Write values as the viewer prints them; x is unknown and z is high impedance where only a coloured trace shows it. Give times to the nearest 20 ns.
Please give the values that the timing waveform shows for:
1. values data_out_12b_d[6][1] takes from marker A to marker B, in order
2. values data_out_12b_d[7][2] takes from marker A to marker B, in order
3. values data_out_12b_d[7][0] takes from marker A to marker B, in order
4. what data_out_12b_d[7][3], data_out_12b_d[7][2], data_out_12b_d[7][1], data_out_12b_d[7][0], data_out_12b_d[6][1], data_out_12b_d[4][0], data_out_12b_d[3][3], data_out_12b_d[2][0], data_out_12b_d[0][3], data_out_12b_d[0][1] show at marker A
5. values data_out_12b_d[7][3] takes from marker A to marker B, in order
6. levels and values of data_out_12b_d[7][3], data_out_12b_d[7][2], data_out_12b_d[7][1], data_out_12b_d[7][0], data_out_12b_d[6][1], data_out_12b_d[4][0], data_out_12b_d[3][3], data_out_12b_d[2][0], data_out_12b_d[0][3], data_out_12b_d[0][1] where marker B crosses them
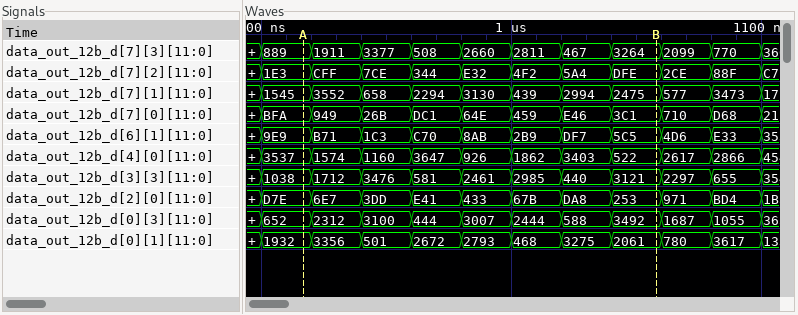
9E9, B71, 1C3, C70, 8AB, 2B9, DF7, 5C5
1E3, CFF, 7CE, 344, E32, 4F2, 5A4, DFE
BFA, 949, 26B, DC1, 64E, 459, E46, 3C1
data_out_12b_d[7][3]=889, data_out_12b_d[7][2]=1E3, data_out_12b_d[7][1]=1545, data_out_12b_d[7][0]=BFA, data_out_12b_d[6][1]=9E9, data_out_12b_d[4][0]=3537, data_out_12b_d[3][3]=1038, data_out_12b_d[2][0]=D7E, data_out_12b_d[0][3]=652, data_out_12b_d[0][1]=1932
889, 1911, 3377, 508, 2660, 2811, 467, 3264
data_out_12b_d[7][3]=3264, data_out_12b_d[7][2]=DFE, data_out_12b_d[7][1]=2475, data_out_12b_d[7][0]=3C1, data_out_12b_d[6][1]=5C5, data_out_12b_d[4][0]=522, data_out_12b_d[3][3]=3121, data_out_12b_d[2][0]=253, data_out_12b_d[0][3]=3492, data_out_12b_d[0][1]=2061
